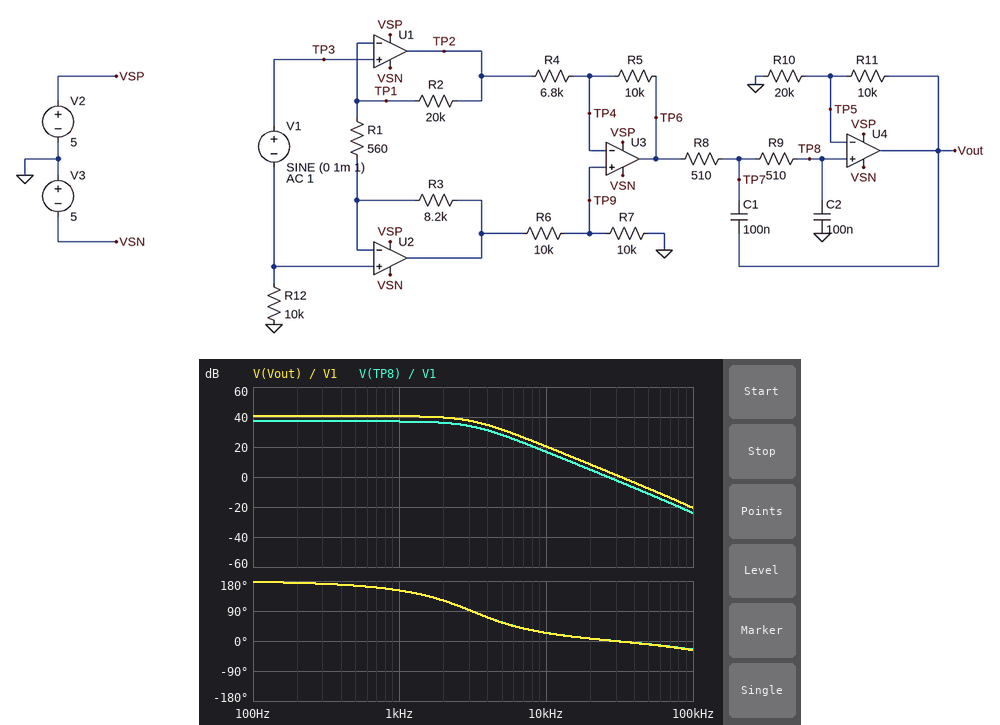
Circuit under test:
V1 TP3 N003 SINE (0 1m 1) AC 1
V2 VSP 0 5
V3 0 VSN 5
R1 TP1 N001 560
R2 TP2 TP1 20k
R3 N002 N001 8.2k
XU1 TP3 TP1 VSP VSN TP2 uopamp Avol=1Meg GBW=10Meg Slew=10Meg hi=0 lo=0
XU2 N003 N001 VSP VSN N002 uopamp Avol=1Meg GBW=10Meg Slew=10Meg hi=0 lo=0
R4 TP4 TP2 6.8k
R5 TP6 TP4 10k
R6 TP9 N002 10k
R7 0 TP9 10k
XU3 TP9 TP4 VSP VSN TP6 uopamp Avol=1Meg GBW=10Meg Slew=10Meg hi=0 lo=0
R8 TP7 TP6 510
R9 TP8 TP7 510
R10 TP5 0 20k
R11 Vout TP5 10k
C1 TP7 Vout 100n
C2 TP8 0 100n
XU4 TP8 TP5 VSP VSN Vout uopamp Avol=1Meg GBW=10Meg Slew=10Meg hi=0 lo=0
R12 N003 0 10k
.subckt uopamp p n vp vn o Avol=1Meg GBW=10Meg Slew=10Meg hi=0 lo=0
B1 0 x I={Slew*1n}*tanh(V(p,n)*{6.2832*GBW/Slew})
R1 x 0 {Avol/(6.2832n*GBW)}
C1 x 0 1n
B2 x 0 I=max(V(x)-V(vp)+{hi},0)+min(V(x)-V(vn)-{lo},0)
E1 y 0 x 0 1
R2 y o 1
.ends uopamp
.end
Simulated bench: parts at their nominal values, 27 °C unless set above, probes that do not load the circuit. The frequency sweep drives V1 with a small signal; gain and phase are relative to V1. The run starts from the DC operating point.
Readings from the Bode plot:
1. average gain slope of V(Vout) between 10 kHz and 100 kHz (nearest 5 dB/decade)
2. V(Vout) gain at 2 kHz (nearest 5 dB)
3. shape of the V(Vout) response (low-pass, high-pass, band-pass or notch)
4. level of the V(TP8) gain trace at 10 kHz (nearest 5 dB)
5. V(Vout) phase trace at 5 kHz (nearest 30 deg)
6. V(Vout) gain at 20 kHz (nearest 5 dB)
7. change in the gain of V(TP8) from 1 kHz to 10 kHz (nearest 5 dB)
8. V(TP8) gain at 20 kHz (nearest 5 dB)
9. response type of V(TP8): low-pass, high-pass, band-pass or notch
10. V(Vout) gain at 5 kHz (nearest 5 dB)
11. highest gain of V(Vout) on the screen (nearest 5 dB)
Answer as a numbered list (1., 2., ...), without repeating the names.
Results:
1. -40 dB/decade
2. 40 dB
3. low-pass
4. 15 dB
5. 60 deg
6. 10 dB
7. -20 dB
8. 5 dB
9. low-pass
10. 30 dB
11. 40 dB
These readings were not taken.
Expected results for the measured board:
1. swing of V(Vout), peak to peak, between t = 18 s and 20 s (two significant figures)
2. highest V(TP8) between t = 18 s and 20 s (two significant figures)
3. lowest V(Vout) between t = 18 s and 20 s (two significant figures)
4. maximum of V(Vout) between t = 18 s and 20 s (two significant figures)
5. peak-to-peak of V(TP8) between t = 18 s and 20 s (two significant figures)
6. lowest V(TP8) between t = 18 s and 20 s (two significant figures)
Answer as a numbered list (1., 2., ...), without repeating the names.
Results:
1. 220 mV
2. 72 mV
3. -110 mV
4. 110 mV
5. 140 mV
6. -72 mV
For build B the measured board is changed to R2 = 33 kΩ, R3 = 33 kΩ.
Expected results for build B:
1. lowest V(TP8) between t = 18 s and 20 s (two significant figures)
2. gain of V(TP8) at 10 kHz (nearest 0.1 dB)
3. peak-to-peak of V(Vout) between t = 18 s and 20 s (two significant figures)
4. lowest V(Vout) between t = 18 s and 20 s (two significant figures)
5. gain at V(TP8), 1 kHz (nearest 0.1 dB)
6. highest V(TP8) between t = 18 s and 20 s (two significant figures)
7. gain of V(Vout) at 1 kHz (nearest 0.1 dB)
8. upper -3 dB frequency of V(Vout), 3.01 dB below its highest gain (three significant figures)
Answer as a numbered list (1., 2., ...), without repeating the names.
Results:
1. -160 mV
2. 23.7 dB
3. 480 mV
4. -240 mV
5. 44.0 dB
6. 160 mV
7. 47.5 dB
8. 2.93 kHz
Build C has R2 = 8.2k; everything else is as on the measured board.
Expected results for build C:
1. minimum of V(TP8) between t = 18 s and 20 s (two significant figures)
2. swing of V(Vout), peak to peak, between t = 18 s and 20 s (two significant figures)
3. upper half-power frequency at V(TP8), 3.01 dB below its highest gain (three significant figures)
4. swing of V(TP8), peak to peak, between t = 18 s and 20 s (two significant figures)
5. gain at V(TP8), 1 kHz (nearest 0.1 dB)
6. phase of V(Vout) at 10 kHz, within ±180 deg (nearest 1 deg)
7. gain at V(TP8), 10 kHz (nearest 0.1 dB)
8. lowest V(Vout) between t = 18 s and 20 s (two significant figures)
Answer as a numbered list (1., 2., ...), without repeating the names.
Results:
1. -41 mV
2. 120 mV
3. 2.93 kHz
4. 82 mV
5. 32.1 dB
6. 25 deg
7. 11.9 dB
8. -62 mV
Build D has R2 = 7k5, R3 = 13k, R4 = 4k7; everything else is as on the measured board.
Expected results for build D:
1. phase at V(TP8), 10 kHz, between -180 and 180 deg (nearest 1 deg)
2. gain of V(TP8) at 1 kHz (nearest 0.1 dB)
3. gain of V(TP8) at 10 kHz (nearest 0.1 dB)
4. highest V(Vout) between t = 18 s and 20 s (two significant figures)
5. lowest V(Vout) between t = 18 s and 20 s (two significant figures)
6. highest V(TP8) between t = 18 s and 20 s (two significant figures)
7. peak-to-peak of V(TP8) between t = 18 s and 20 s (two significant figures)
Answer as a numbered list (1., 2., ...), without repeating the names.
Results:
1. 25 deg
2. 36.4 dB
3. 16.1 dB
4. 100 mV
5. -100 mV
6. 67 mV
7. 130 mV
